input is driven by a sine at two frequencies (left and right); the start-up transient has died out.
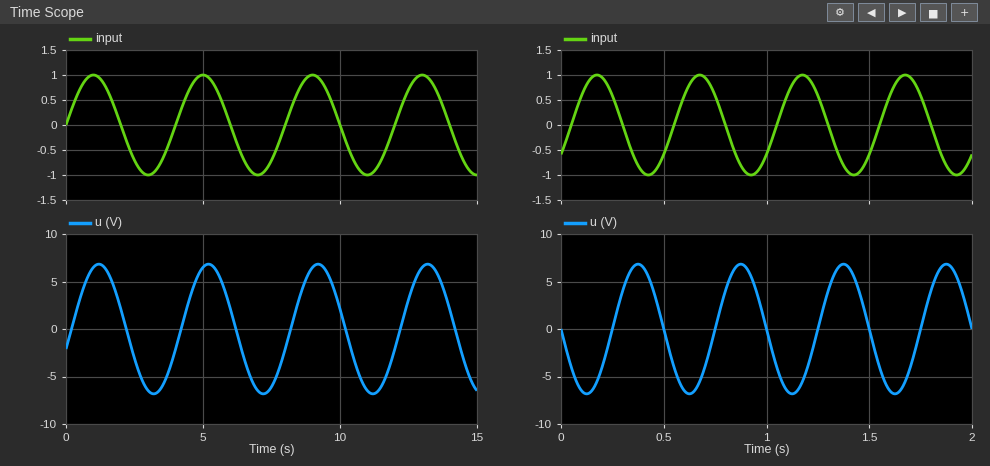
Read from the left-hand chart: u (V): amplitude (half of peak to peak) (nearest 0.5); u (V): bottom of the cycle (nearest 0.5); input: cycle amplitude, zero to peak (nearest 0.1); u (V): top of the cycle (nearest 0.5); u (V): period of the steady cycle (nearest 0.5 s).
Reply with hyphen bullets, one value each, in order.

- 7.0
- -7.0
- 1.0
- 7.0
- 4.0 s
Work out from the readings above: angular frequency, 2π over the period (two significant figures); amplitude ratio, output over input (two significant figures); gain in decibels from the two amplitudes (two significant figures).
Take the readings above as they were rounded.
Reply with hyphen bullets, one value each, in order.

- 1.6 rad/s
- 7.0
- 17 dB
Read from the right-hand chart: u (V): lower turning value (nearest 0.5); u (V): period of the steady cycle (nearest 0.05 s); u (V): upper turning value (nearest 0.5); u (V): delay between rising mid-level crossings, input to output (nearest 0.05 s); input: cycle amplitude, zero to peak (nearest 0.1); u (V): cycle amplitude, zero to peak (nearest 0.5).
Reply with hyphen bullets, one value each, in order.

- -7.0
- 0.50 s
- 7.0
- 0.20 s
- 1.0
- 7.0
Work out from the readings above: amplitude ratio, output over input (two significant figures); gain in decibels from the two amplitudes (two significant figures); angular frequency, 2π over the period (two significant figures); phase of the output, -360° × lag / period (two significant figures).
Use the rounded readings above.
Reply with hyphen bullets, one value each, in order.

- 7.0
- 17 dB
- 13 rad/s
- -140°
